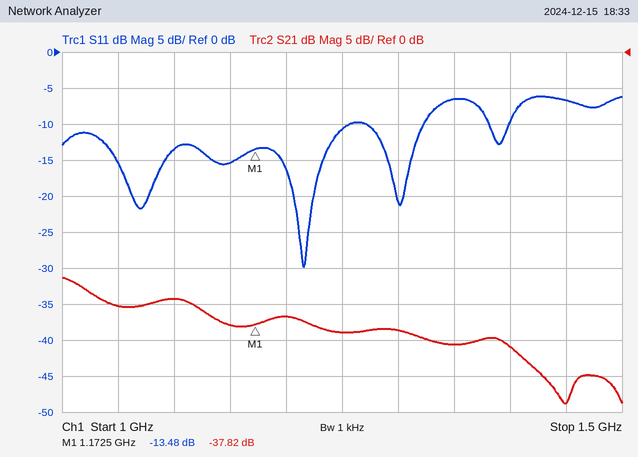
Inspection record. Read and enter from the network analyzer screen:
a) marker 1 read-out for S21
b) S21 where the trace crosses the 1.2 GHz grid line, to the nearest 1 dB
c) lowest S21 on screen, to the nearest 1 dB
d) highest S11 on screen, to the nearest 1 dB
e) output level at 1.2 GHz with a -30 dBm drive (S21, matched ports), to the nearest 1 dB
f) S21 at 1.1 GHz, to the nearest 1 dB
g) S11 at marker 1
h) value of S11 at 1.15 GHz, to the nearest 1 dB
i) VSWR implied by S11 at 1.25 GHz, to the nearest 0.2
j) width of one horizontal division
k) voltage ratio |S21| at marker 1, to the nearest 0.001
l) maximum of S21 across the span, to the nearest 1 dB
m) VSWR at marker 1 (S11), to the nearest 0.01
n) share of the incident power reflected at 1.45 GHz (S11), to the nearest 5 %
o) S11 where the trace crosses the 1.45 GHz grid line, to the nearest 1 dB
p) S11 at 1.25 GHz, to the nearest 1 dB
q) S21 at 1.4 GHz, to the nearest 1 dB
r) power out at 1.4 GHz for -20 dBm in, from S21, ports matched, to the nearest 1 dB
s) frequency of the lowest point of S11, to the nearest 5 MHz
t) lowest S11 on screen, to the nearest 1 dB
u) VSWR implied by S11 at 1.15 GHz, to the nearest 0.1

-37.82 dB
-37 dB
-49 dB
-6 dB
-67 dBm
-34 dB
-13.48 dB
-15 dB
1.8
50 MHz
0.013
-31 dB
1.54
20 %
-7 dB
-11 dB
-41 dB
-61 dBm
1.215 GHz
-30 dB
1.4
